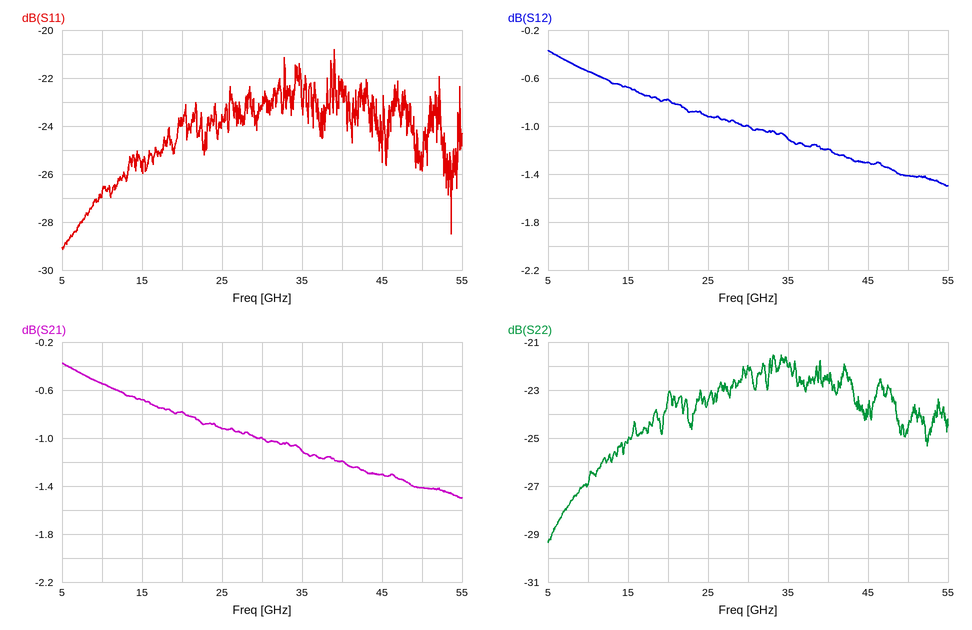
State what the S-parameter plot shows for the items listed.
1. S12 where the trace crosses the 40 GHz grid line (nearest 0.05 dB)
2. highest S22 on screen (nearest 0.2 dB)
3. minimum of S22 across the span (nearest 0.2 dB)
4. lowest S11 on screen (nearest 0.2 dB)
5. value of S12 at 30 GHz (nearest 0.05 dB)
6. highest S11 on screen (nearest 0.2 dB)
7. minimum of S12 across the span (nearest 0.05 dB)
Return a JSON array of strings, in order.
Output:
["-1.20 dB", "-21.6 dB", "-29.4 dB", "-29.2 dB", "-1.00 dB", "-20.8 dB", "-1.50 dB"]
